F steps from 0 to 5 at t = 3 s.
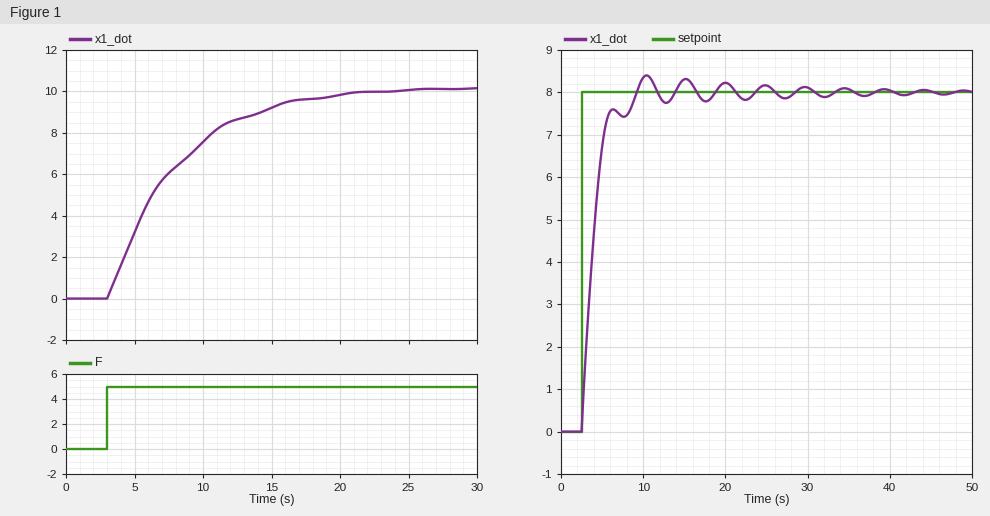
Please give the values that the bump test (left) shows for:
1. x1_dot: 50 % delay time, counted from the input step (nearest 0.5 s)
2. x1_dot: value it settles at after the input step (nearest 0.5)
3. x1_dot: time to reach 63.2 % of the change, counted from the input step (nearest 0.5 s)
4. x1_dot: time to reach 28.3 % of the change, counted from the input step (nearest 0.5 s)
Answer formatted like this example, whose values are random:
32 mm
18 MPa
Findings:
3.5 s
10.0
5.0 s
2.0 s
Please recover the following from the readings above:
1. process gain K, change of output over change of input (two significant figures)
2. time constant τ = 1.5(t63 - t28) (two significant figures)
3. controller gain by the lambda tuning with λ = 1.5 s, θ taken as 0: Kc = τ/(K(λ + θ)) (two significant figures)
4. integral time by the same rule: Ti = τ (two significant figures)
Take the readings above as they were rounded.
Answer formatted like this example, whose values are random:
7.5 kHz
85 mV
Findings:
2.0
4.5 s
1.5
4.5 s
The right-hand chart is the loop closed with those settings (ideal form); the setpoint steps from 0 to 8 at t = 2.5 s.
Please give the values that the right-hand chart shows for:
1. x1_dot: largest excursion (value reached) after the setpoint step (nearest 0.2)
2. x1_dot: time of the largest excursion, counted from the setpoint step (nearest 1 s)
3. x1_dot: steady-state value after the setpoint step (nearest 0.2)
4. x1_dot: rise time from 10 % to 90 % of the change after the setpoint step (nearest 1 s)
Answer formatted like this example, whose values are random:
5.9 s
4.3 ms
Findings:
8.4
8 s
8.0
3 s
